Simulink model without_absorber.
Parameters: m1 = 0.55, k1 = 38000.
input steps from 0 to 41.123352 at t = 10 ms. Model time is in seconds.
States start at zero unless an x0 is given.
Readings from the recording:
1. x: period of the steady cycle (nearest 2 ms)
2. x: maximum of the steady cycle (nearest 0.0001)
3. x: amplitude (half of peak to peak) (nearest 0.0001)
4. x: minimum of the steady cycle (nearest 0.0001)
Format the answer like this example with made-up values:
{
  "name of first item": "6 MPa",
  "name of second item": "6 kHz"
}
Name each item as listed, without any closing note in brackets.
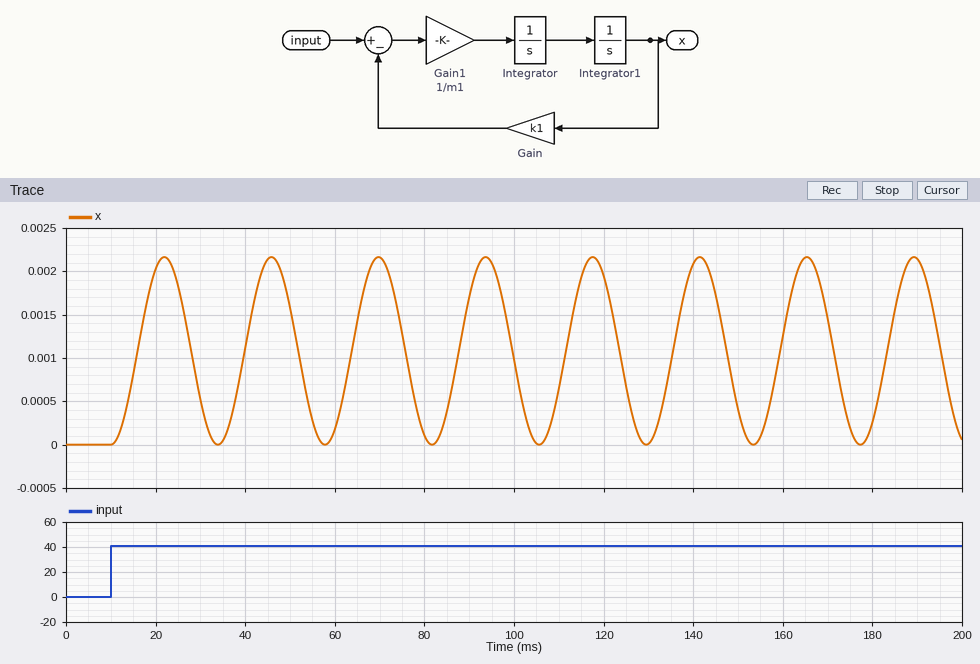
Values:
{
  "x: period of the steady cycle": "24 ms",
  "x: maximum of the steady cycle": "0.0022",
  "x: amplitude (half of peak to peak)": "0.0011",
  "x: minimum of the steady cycle": "0.0000"
}
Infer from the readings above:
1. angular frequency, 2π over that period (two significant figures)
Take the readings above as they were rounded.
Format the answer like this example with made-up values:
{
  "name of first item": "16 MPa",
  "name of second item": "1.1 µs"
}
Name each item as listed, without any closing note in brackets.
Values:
{
  "angular frequency, 2π over that period": "0.26 rad/ms"
}
